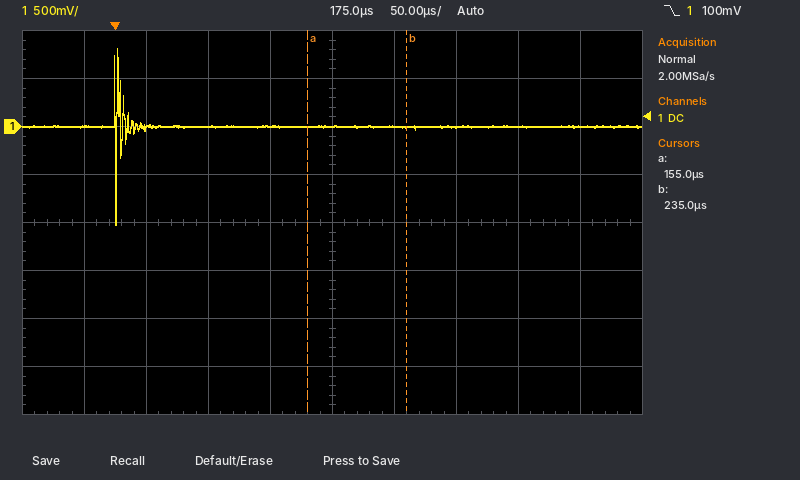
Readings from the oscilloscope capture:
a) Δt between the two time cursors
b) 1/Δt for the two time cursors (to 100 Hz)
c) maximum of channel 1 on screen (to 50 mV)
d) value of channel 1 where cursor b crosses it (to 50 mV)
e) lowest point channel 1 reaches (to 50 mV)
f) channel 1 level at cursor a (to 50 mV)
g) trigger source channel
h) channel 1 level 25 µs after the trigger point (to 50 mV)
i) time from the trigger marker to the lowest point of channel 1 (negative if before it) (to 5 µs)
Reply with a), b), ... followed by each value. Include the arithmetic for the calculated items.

a) 235 µs − (155 µs) = 80 µs
b) 1 / 80 µs ≈ 12.5 kHz
c) 800 mV
d) 0 mV
e) -1.00 V
f) 0 mV
g) channel 1
h) 0 mV
i) 0 µs
